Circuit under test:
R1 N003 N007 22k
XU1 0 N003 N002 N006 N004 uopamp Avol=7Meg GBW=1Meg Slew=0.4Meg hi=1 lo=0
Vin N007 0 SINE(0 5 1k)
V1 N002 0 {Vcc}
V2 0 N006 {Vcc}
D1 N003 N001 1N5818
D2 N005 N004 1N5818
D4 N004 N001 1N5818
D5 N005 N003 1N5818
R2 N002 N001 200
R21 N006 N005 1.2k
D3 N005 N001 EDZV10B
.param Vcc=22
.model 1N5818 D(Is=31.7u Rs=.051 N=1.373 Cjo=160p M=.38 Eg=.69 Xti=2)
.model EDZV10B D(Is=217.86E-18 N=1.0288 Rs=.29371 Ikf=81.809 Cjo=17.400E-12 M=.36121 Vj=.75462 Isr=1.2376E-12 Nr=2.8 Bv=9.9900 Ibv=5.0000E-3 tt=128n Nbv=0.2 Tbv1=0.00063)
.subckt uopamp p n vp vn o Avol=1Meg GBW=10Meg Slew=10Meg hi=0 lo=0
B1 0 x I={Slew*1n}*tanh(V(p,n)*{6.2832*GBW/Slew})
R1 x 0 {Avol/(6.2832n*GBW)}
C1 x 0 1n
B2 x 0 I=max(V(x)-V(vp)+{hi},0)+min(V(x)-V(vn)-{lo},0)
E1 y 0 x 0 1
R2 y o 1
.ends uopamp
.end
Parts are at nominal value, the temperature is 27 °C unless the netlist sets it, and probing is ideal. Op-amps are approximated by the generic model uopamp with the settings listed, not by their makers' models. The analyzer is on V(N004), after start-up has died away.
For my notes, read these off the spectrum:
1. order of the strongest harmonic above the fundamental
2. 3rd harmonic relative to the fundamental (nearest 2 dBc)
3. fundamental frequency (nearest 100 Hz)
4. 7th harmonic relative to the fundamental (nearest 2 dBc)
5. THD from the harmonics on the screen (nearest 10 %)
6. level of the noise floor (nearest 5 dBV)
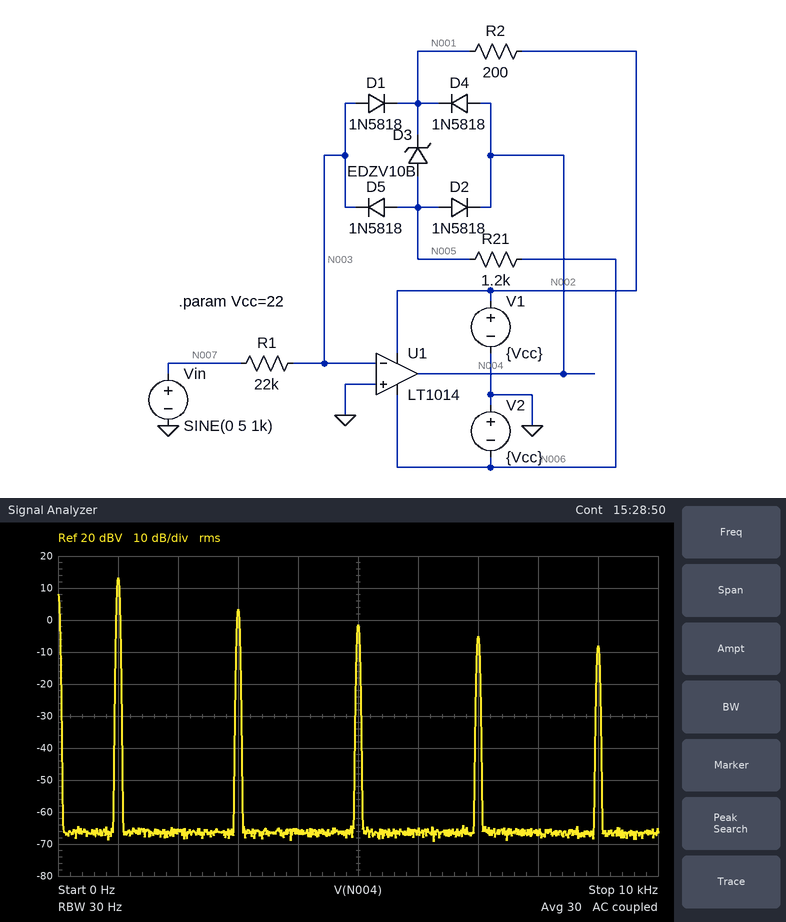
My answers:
3
-10 dBc
1.0 kHz
-18 dBc
40 %
-65 dBV
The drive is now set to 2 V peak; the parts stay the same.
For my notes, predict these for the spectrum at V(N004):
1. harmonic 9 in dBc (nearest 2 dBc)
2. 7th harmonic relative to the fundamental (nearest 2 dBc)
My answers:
-24 dBc
-20 dBc
